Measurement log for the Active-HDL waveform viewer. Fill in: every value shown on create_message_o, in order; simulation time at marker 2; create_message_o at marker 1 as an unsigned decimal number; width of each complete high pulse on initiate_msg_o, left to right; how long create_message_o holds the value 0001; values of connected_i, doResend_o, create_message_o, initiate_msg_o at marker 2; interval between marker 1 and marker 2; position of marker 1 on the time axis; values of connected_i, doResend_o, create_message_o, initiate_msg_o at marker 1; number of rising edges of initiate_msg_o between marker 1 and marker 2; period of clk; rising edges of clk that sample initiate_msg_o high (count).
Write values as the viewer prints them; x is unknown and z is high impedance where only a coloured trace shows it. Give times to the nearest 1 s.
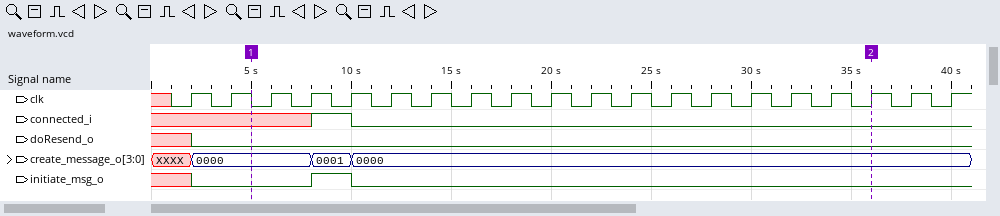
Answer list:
XXXX, 0000, 0001, 0000
36 s
0
2 s
2 s
connected_i=0, doResend_o=0, create_message_o=0000, initiate_msg_o=0
31 s
5 s
connected_i=x, doResend_o=0, create_message_o=0000, initiate_msg_o=0
1
2 s
1
